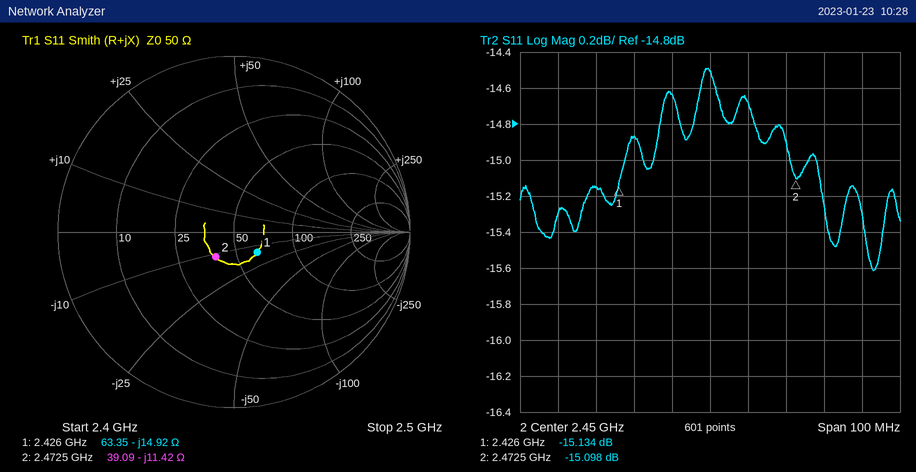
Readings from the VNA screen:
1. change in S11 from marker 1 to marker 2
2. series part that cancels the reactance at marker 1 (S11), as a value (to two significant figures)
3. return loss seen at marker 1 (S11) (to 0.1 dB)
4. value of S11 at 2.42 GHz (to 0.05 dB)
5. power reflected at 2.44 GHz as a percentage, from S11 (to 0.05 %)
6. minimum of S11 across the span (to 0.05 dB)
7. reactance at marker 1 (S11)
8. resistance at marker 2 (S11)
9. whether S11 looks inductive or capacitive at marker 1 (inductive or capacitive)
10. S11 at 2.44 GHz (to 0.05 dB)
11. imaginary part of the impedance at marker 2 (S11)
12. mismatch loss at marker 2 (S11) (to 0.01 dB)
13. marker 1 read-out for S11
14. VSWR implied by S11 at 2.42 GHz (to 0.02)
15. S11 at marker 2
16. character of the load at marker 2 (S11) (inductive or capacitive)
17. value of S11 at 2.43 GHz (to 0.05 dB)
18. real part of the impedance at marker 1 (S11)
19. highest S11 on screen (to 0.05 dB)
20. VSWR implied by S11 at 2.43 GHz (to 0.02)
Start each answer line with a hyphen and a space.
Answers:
- 0.036 dB
- 980 pH
- 15.1 dB
- -15.15 dB
- 3.45 %
- -15.60 dB
- -14.92 Ω
- 39.09 Ω
- capacitive
- -14.65 dB
- -11.42 Ω
- 0.14 dB
- -15.134 dB
- 1.42
- -15.098 dB
- capacitive
- -14.85 dB
- 63.35 Ω
- -14.50 dB
- 1.44
